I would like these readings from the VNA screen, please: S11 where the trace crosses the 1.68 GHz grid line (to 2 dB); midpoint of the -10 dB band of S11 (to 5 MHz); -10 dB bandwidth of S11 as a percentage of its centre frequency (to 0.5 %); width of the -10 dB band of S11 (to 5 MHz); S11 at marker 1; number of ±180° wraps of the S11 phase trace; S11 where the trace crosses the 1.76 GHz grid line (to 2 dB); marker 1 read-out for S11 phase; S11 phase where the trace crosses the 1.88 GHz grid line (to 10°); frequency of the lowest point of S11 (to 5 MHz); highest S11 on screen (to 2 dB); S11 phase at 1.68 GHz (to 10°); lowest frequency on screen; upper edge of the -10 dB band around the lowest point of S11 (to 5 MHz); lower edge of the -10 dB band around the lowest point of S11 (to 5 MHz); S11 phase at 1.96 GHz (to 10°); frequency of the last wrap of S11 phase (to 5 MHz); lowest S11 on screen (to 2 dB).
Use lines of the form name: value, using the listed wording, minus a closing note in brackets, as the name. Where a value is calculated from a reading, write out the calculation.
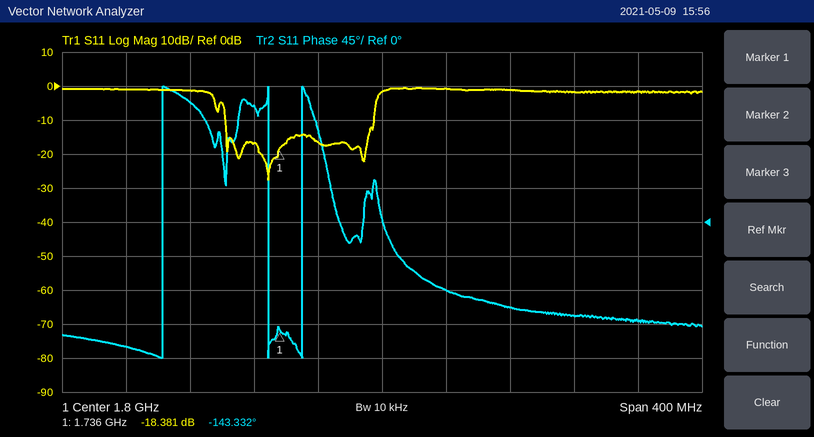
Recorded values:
S11 where the trace crosses the 1.68 GHz grid line: -2 dB
midpoint of the -10 dB band of S11: 1.750 GHz
-10 dB bandwidth of S11 as a percentage of its centre frequency: 95 MHz / 1.7475 GHz ≈ 5.44 %, so 5.5 % to the nearest 0.5 %
width of the -10 dB band of S11: 1.795 GHz − 1.700 GHz = 95 MHz
S11 at marker 1: -18.381 dB
number of ±180° wraps of the S11 phase trace: 3
S11 where the trace crosses the 1.76 GHz grid line: -16 dB
marker 1 read-out for S11 phase: -143.332°
S11 phase where the trace crosses the 1.88 GHz grid line: -110°
frequency of the lowest point of S11: 1.730 GHz
highest S11 on screen: 0 dB
S11 phase at 1.68 GHz: 160°
lowest frequency on screen: 1.6 GHz
upper edge of the -10 dB band around the lowest point of S11: 1.795 GHz
lower edge of the -10 dB band around the lowest point of S11: 1.700 GHz
S11 phase at 1.96 GHz: -130°
frequency of the last wrap of S11 phase: 1.750 GHz
lowest S11 on screen: -28 dB
